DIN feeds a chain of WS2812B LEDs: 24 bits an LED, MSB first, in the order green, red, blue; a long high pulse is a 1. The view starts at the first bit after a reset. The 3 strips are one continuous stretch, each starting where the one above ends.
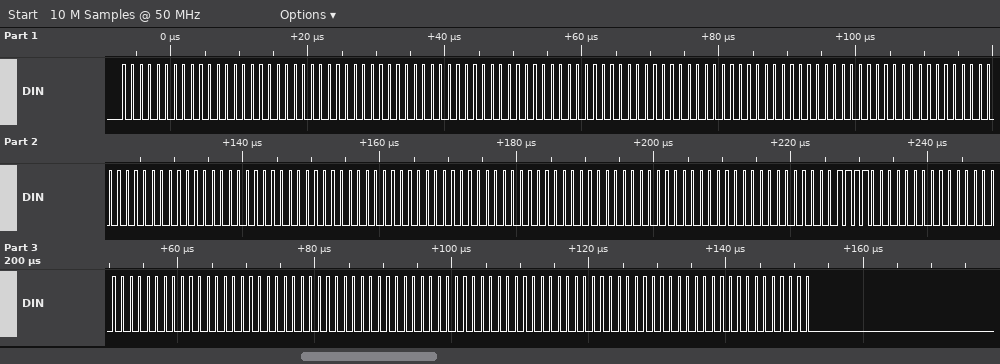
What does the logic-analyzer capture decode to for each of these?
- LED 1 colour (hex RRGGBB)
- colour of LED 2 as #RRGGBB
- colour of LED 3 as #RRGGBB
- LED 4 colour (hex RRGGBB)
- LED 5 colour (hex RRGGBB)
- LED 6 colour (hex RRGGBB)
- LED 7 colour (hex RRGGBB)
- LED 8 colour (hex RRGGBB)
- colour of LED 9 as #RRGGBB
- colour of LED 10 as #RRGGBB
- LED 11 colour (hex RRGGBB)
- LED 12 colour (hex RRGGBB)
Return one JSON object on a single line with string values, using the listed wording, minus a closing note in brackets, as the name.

{"LED 1 colour": "#000000", "colour of LED 2 as #RRGGBB": "#000000", "colour of LED 3 as #RRGGBB": "#000000", "LED 4 colour": "#000000", "LED 5 colour": "#000000", "LED 6 colour": "#000000", "LED 7 colour": "#000000", "LED 8 colour": "#00001E", "colour of LED 9 as #RRGGBB": "#000000", "colour of LED 10 as #RRGGBB": "#000000", "LED 11 colour": "#000000", "LED 12 colour": "#000000"}
